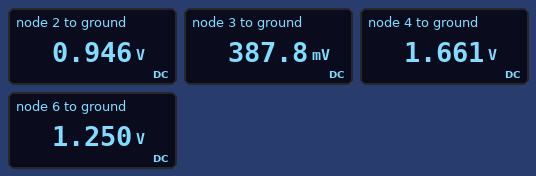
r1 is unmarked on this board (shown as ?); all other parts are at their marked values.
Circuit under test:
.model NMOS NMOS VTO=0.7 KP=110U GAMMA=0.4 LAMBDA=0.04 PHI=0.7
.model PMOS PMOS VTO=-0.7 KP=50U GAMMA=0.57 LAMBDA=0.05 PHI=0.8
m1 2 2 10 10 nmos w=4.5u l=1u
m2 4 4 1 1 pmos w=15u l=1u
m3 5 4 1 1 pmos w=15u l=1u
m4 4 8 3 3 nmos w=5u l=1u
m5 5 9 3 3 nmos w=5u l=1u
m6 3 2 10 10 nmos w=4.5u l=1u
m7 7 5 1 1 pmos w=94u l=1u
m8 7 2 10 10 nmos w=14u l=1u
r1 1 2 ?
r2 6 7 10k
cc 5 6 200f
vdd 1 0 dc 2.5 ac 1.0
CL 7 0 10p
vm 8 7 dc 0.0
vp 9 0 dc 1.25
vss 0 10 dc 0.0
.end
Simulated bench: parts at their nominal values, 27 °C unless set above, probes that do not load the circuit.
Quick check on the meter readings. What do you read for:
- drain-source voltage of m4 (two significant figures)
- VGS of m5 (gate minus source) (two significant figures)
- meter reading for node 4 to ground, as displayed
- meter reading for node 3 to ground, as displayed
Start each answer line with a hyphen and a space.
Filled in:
- 1.3 V
- 860 mV
- 1.661 V
- 387.8 mV
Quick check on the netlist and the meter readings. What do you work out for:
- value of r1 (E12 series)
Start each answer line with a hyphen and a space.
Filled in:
- 100 kΩ
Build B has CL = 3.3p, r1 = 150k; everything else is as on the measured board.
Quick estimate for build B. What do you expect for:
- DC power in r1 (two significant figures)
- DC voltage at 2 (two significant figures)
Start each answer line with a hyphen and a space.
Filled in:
- 17 µW
- 900 mV
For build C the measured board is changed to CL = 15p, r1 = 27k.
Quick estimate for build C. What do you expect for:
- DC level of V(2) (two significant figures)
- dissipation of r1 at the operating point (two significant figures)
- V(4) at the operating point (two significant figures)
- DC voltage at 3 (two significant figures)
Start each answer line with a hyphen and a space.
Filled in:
- 1.1 V
- 68 µW
- 1.6 V
- 280 mV
